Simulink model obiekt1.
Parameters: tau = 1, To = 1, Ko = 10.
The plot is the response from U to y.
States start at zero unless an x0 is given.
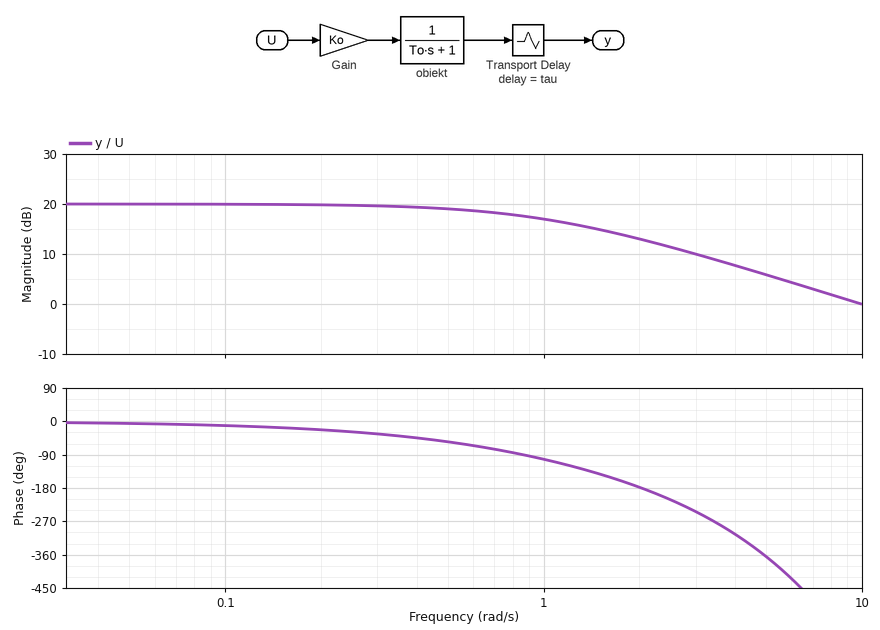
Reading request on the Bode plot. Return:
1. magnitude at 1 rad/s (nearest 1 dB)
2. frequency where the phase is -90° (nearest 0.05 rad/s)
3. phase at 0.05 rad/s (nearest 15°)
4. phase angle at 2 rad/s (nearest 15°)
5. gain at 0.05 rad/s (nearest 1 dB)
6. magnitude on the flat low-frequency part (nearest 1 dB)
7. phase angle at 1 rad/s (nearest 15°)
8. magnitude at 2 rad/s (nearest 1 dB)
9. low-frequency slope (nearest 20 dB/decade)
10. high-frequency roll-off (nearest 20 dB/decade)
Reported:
17 dB
0.85 rad/s
0°
-180°
20 dB
20 dB
-105°
13 dB
0 dB/decade
-20 dB/decade
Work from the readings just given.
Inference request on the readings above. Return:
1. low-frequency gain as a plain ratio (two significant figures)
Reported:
10
